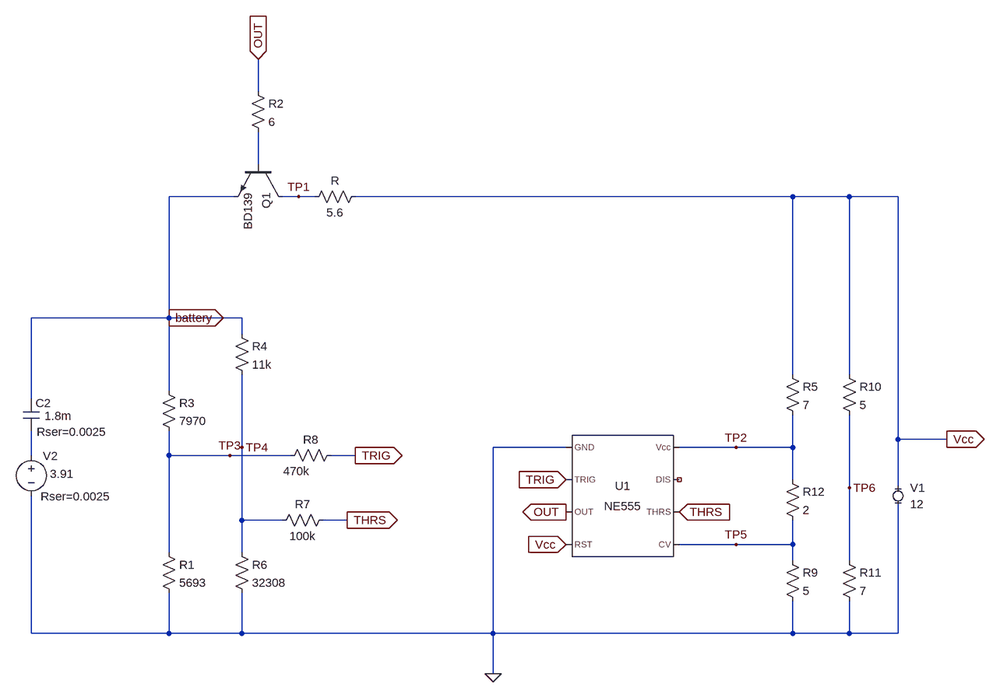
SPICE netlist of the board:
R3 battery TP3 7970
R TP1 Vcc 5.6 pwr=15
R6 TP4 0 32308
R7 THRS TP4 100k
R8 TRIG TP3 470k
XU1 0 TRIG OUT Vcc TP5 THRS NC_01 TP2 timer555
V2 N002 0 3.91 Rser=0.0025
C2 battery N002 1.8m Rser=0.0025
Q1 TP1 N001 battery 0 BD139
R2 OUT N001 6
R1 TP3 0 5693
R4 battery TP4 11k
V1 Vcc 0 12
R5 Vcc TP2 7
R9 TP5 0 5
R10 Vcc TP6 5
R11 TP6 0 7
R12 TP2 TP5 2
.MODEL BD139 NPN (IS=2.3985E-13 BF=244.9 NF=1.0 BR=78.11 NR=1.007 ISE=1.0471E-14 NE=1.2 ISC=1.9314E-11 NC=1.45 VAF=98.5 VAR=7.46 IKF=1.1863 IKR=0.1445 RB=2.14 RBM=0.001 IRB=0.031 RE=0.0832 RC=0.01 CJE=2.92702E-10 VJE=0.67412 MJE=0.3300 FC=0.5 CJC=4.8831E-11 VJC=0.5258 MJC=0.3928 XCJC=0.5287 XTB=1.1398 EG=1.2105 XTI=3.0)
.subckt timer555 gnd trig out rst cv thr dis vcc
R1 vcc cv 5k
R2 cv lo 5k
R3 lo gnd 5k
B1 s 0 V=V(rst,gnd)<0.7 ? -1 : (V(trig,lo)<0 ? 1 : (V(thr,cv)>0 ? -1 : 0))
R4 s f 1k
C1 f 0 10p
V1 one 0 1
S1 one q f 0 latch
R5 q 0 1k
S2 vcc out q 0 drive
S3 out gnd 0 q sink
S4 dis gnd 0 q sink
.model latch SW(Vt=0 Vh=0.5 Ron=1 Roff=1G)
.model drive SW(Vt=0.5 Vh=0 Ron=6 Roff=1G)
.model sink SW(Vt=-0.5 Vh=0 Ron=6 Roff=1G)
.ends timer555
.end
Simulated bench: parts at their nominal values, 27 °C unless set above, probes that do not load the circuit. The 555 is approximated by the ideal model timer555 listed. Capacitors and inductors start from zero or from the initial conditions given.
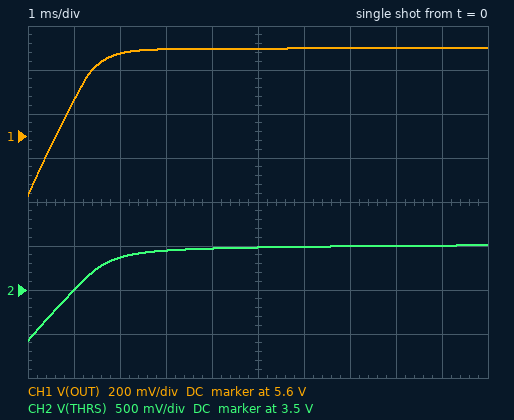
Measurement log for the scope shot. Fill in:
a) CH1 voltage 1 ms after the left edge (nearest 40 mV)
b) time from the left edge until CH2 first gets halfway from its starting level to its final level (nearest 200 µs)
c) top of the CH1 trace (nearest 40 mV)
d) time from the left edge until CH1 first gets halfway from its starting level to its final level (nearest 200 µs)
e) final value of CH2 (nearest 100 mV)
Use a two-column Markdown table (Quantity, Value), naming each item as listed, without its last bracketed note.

| Quantity | Value |
|---|---|
| CH1 voltage 1 ms after the left edge | 5.76 V |
| time from the left edge until CH2 first gets halfway from its starting level to its final level | 1.0 ms |
| top of the CH1 trace | 6.00 V |
| time from the left edge until CH1 first gets halfway from its starting level to its final level | 800 µs |
| final value of CH2 | 4.0 V |
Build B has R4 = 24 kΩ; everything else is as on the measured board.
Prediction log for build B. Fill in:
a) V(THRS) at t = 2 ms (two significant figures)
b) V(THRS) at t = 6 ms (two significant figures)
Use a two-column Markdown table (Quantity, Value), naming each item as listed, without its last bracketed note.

| Quantity | Value |
|---|---|
| V(THRS) at t = 2 ms | 3.0 V |
| V(THRS) at t = 6 ms | 3.1 V |
